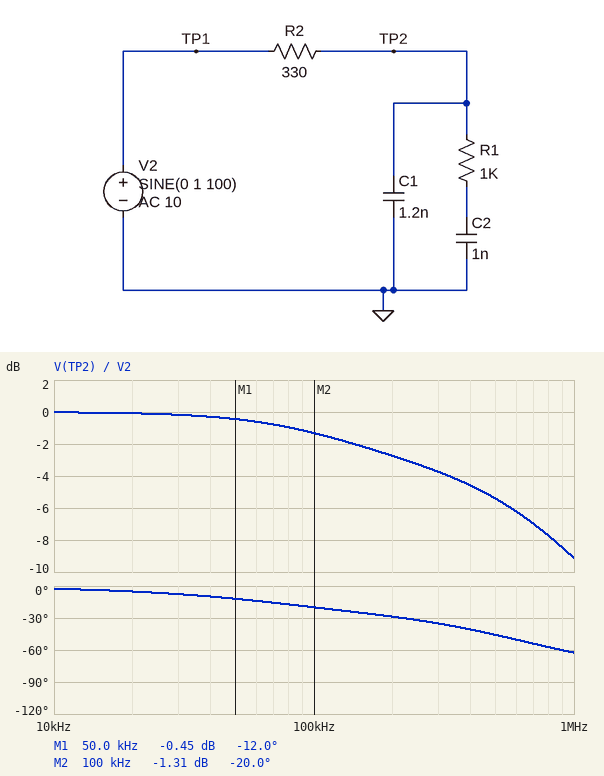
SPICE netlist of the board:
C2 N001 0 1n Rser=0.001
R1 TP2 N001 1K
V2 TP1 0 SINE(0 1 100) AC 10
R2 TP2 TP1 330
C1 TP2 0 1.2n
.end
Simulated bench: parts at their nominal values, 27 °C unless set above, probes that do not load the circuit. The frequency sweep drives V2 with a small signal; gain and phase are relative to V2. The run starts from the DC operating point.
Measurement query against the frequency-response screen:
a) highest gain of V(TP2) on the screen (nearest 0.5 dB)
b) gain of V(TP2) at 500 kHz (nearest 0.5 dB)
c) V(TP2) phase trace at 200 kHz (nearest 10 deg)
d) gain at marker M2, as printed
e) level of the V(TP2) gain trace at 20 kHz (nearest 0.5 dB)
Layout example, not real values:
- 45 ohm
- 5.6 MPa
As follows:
- 0 dB
- -5.5 dB
- -30 deg
- -1.31 dB
- 0 dB
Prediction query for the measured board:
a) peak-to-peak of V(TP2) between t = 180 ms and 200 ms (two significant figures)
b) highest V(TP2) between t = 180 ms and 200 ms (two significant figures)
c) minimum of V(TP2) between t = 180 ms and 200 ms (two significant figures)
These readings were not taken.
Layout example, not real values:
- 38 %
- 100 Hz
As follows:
- 2.0 V
- 1.0 V
- -1.0 V
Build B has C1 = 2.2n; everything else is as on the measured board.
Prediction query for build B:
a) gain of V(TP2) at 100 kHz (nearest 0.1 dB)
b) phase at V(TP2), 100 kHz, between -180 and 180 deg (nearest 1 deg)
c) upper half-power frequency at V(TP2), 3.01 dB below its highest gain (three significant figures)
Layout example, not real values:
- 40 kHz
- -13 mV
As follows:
- -1.9 dB
- -29 deg
- 145 kHz
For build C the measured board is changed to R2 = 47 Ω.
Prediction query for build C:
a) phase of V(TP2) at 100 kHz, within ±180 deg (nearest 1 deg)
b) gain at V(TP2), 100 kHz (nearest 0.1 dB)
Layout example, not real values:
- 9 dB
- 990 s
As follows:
- -3 deg
- -0.1 dB
